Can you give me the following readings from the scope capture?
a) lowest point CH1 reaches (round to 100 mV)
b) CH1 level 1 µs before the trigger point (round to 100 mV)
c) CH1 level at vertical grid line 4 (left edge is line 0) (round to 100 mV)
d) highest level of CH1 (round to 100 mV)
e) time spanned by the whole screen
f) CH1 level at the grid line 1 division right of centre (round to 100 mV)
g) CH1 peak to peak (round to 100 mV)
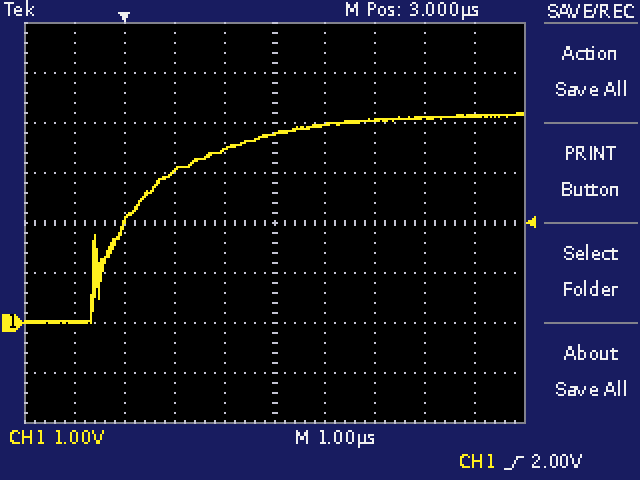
0.0 V
0.0 V
3.5 V
4.2 V
10 µs
4.0 V
4.2 V
